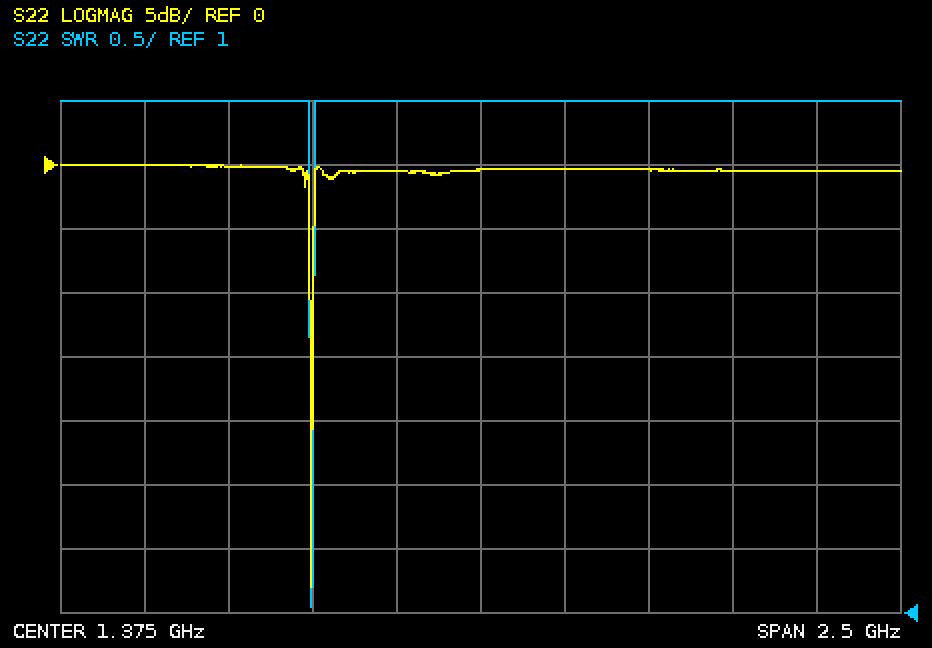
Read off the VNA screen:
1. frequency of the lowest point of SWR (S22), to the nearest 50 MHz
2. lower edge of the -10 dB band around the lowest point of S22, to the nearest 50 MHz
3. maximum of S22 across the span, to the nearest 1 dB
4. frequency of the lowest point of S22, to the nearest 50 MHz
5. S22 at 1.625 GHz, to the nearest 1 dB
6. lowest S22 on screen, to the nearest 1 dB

850 MHz
850 MHz
0 dB
850 MHz
0 dB
-33 dB
